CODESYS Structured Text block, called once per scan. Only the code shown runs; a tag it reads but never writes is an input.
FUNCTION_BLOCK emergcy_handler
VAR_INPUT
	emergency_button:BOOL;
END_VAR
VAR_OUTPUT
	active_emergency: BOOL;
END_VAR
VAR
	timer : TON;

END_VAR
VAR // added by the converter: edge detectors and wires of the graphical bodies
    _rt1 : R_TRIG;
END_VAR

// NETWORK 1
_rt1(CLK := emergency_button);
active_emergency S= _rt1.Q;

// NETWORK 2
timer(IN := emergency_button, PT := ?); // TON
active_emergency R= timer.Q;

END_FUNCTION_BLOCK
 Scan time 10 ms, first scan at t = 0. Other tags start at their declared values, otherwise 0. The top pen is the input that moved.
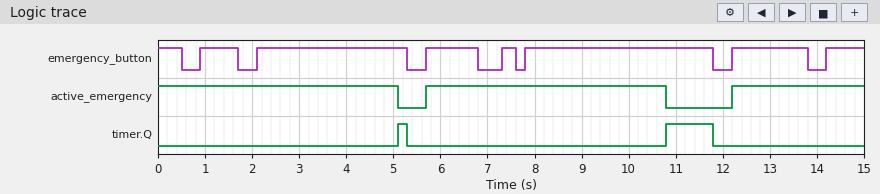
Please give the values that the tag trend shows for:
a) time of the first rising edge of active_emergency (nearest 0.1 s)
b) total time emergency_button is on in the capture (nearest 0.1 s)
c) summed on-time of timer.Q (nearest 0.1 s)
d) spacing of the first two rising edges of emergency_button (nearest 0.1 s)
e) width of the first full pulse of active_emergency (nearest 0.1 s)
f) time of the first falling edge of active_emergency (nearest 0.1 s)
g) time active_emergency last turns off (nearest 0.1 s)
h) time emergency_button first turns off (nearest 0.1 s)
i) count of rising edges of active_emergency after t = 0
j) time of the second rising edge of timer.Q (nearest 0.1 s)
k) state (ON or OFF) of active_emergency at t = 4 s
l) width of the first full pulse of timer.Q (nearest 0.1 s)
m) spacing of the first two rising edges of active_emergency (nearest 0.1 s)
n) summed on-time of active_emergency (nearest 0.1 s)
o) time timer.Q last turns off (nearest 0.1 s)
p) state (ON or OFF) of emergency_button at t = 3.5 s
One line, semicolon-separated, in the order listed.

5.7 s; 12.3 s; 1.2 s; 1.2 s; 5.1 s; 5.1 s; 10.8 s; 0.5 s; 2; 10.8 s; ON; 0.2 s; 6.5 s; 13.0 s; 11.8 s; ON
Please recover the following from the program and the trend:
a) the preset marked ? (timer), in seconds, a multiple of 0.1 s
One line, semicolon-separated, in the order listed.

3.0 s
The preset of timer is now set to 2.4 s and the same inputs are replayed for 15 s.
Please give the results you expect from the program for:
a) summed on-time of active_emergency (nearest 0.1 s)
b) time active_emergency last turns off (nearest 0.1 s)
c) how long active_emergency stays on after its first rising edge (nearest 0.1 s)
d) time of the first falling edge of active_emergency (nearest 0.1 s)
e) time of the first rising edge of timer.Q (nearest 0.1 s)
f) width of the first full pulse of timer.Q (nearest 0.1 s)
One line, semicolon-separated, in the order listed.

11.8 s; 10.2 s; 4.5 s; 4.5 s; 4.5 s; 0.8 s
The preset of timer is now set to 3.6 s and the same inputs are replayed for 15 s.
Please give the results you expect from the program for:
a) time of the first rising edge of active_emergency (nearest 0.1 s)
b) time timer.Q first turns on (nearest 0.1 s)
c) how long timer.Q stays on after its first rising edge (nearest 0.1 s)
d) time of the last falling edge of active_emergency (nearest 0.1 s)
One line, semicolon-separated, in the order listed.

12.2 s; 11.4 s; 0.4 s; 11.4 s
